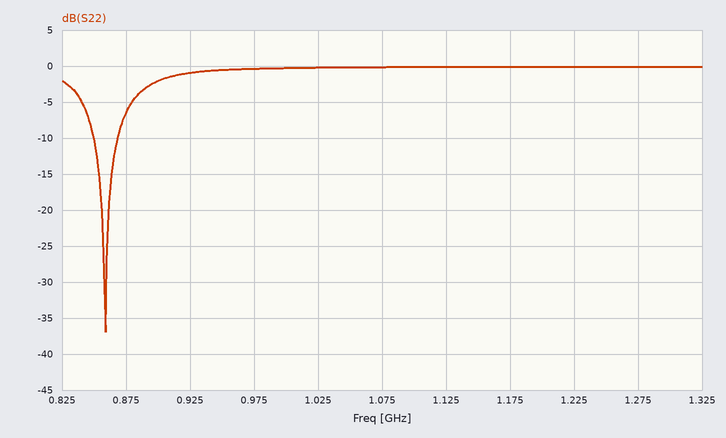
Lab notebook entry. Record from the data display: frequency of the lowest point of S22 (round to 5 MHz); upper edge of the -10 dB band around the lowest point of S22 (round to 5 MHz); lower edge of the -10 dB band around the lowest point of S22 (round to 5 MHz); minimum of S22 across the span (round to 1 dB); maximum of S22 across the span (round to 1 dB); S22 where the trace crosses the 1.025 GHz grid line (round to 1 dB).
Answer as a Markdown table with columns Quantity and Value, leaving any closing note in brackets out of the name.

| Quantity | Value |
|---|---|
| frequency of the lowest point of S22 | 860 MHz |
| upper edge of the -10 dB band around the lowest point of S22 | 870 MHz |
| lower edge of the -10 dB band around the lowest point of S22 | 850 MHz |
| minimum of S22 across the span | -37 dB |
| maximum of S22 across the span | 0 dB |
| S22 where the trace crosses the 1.025 GHz grid line | 0 dB |
